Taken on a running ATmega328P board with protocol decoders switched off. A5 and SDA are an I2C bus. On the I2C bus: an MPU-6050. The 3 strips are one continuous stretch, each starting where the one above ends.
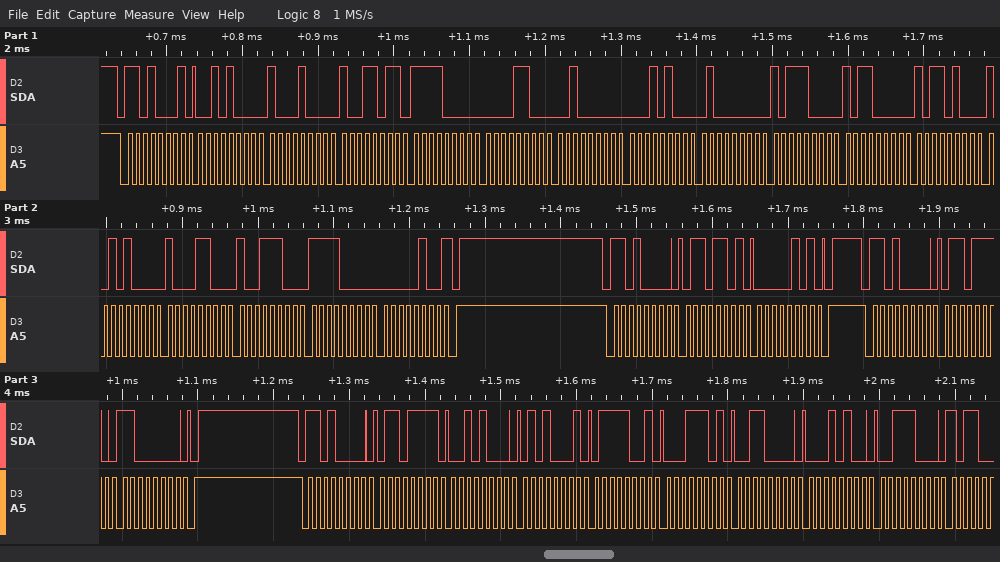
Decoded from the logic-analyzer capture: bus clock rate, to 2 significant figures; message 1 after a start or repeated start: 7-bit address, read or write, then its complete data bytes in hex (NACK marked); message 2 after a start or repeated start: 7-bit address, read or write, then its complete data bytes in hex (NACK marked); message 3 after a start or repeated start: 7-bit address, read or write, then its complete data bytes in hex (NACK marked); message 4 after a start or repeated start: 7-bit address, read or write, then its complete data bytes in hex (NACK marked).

100 kHz
0x68 read: 28 88 9B F0 0C 20 14 40 B8 B0 B4 A8 8C 9C F0 04 NACK
0x68 write: 6D 05
0x68 write: 6E C0
0x68 write: 6F 28 51 79 1D 30 14 38
